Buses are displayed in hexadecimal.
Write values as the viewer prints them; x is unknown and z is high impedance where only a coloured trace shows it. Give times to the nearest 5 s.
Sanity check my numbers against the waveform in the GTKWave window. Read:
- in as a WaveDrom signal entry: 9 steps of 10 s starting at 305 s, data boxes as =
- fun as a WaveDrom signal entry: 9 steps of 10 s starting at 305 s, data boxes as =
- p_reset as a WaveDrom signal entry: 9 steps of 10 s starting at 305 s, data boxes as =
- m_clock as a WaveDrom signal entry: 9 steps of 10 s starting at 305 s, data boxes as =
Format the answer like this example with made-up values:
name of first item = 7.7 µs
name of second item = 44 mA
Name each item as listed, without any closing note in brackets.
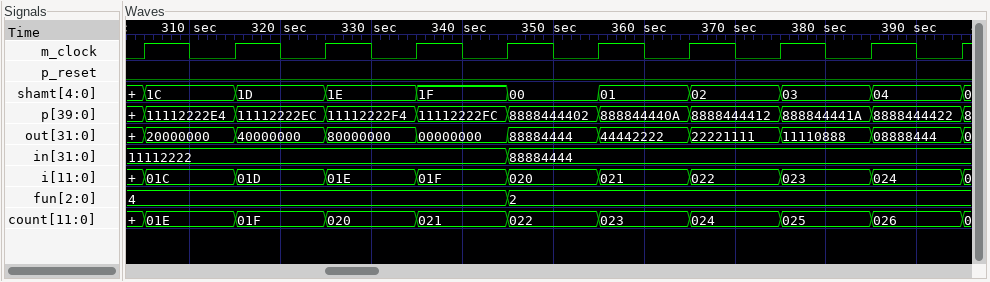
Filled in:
in as a WaveDrom signal entry: 9 steps of 10 s starting at 305 s, data boxes as = = {name: 'in', wave: '=...=....', data: '11112222 88884444'}
fun as a WaveDrom signal entry: 9 steps of 10 s starting at 305 s, data boxes as = = {name: 'fun', wave: '=...=....', data: '4 2'}
p_reset as a WaveDrom signal entry: 9 steps of 10 s starting at 305 s, data boxes as = = {name: 'p_reset', wave: '0........'}
m_clock as a WaveDrom signal entry: 9 steps of 10 s starting at 305 s, data boxes as = = {name: 'm_clock', wave: 'p........'}
